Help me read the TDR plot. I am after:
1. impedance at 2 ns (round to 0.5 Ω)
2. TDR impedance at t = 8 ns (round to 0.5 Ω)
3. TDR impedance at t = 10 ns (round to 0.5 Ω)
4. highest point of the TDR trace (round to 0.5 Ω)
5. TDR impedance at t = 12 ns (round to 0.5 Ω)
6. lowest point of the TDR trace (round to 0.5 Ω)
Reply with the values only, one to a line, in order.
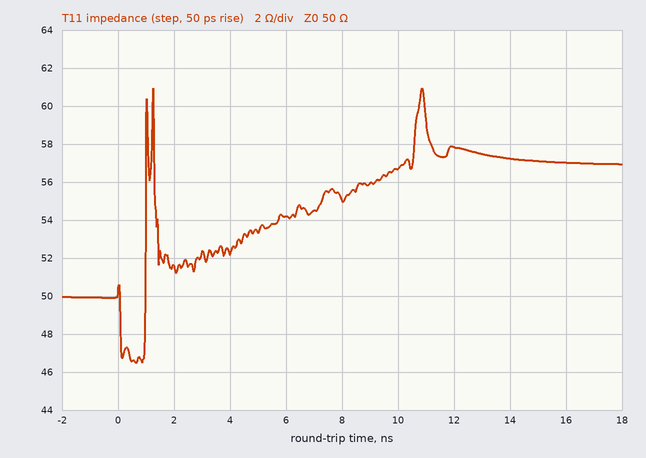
51.5 Ω
55.0 Ω
56.5 Ω
61.0 Ω
58.0 Ω
46.5 Ω
